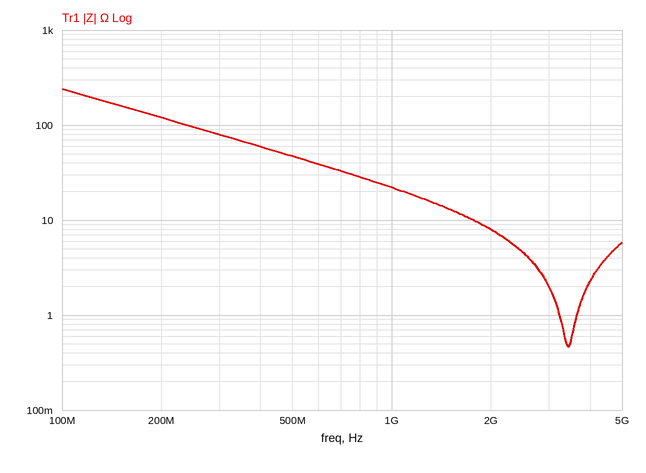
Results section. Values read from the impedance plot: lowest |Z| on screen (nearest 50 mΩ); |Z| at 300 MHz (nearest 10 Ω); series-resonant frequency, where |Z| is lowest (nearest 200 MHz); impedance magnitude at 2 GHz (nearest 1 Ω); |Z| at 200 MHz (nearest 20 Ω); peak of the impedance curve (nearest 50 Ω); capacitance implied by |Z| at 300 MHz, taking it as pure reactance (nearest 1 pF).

450 mΩ
80 Ω
3.4 GHz
8 Ω
120 Ω
250 Ω
7 pF
